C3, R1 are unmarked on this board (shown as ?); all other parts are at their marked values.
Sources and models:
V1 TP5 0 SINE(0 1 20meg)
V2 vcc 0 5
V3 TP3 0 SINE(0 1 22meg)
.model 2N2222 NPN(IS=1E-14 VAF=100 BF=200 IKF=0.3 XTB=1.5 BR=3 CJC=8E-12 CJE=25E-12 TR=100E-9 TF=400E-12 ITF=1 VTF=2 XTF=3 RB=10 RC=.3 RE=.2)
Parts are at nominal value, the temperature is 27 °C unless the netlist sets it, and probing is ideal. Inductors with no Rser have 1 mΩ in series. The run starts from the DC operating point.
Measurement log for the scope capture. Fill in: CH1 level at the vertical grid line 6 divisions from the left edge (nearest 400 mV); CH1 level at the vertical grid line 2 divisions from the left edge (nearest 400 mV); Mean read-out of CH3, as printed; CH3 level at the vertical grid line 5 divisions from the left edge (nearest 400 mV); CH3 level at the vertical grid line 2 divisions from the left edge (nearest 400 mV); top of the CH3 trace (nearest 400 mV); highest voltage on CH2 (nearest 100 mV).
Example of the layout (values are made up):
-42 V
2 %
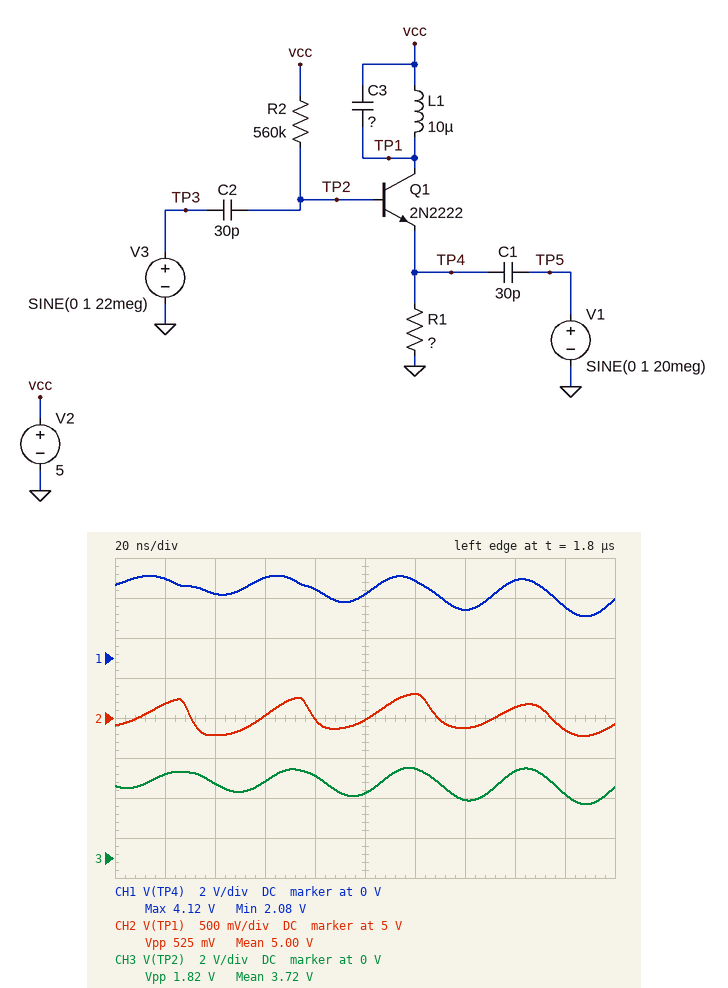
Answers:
4.0 V
3.2 V
3.72 V
3.2 V
3.6 V
4.4 V
5.3 V
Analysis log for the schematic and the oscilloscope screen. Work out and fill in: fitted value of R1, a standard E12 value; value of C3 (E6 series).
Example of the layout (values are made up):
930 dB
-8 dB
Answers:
5.6 kΩ
47 pF
